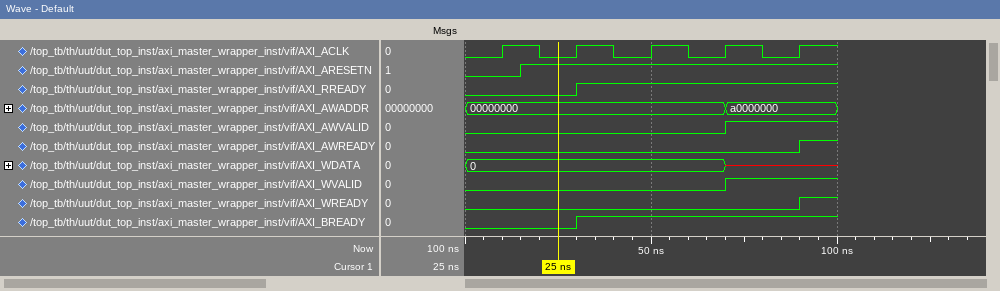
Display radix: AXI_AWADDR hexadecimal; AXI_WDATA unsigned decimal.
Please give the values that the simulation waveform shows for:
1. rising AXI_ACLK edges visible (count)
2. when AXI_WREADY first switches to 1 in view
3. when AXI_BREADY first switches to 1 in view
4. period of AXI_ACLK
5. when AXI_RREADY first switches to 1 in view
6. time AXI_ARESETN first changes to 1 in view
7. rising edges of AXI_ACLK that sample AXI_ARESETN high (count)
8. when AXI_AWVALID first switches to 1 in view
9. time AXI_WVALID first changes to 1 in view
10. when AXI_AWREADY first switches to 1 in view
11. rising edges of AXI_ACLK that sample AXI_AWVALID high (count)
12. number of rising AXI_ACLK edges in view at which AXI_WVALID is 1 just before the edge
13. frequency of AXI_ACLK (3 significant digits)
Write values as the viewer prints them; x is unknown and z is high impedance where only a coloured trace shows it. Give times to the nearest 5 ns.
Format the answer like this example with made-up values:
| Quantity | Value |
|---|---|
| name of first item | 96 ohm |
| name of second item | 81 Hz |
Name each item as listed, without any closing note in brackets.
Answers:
| Quantity | Value |
|---|---|
| rising AXI_ACLK edges visible | 5 |
| when AXI_WREADY first switches to 1 in view | 90 ns |
| when AXI_BREADY first switches to 1 in view | 30 ns |
| period of AXI_ACLK | 20 ns |
| when AXI_RREADY first switches to 1 in view | 30 ns |
| time AXI_ARESETN first changes to 1 in view | 15 ns |
| rising edges of AXI_ACLK that sample AXI_ARESETN high | 4 |
| when AXI_AWVALID first switches to 1 in view | 70 ns |
| time AXI_WVALID first changes to 1 in view | 70 ns |
| when AXI_AWREADY first switches to 1 in view | 90 ns |
| rising edges of AXI_ACLK that sample AXI_AWVALID high | 1 |
| number of rising AXI_ACLK edges in view at which AXI_WVALID is 1 just before the edge | 1 |
| frequency of AXI_ACLK | 50.0 MHz |
